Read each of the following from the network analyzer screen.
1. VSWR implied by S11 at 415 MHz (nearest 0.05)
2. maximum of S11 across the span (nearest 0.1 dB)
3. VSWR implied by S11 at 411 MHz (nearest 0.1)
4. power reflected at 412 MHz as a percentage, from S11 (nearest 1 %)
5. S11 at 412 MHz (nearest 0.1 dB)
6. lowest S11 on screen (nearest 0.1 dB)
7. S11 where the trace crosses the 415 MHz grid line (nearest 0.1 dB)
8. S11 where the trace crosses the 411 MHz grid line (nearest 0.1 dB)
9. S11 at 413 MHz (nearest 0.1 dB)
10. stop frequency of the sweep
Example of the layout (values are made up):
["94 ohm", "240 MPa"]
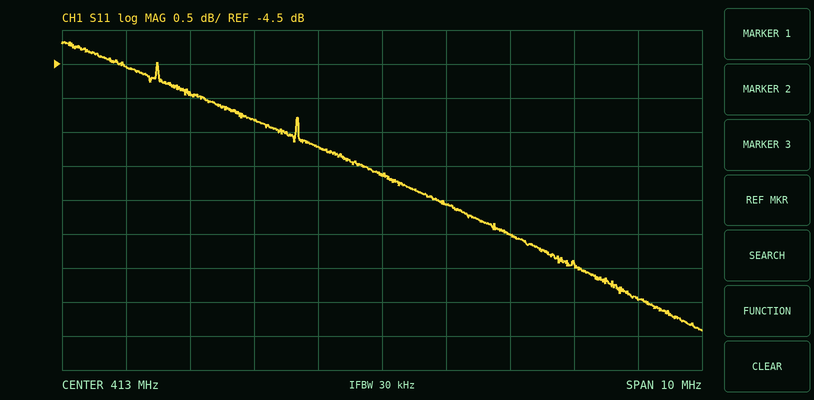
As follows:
["2.60", "-4.2 dB", "3.4", "27 %", "-5.7 dB", "-8.4 dB", "-7.0 dB", "-5.3 dB", "-6.1 dB", "418 MHz"]
